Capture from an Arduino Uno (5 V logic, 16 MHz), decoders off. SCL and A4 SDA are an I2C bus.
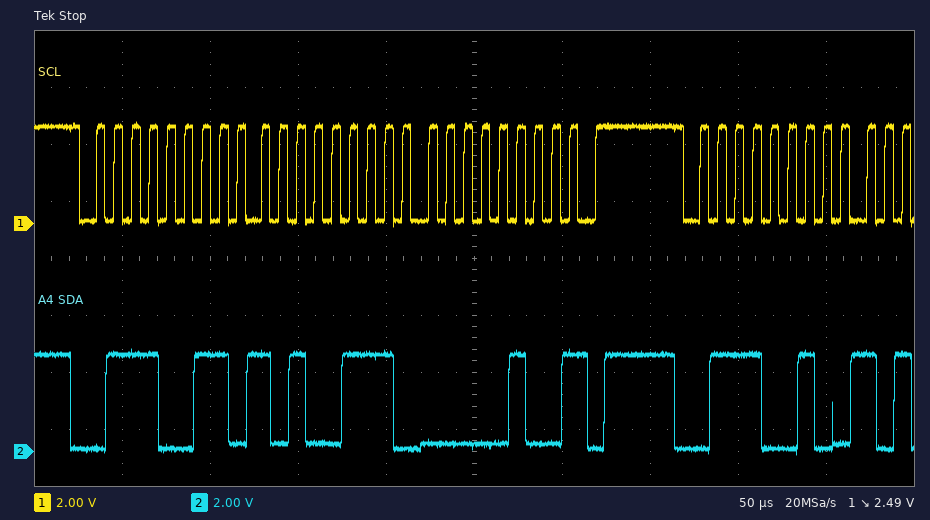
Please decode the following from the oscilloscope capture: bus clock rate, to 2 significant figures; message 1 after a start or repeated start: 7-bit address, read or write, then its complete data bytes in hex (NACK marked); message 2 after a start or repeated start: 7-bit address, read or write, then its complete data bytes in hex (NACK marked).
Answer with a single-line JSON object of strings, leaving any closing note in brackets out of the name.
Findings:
{"bus clock rate, to 2 significant figures": "100 kHz", "message 1 after a start or repeated start: 7-bit address, read or write, then its complete data bytes in hex": "0x39 read: A7 04 NACK", "message 2 after a start or repeated start: 7-bit address, read or write, then its complete data bytes in hex": "0x39 write"}
